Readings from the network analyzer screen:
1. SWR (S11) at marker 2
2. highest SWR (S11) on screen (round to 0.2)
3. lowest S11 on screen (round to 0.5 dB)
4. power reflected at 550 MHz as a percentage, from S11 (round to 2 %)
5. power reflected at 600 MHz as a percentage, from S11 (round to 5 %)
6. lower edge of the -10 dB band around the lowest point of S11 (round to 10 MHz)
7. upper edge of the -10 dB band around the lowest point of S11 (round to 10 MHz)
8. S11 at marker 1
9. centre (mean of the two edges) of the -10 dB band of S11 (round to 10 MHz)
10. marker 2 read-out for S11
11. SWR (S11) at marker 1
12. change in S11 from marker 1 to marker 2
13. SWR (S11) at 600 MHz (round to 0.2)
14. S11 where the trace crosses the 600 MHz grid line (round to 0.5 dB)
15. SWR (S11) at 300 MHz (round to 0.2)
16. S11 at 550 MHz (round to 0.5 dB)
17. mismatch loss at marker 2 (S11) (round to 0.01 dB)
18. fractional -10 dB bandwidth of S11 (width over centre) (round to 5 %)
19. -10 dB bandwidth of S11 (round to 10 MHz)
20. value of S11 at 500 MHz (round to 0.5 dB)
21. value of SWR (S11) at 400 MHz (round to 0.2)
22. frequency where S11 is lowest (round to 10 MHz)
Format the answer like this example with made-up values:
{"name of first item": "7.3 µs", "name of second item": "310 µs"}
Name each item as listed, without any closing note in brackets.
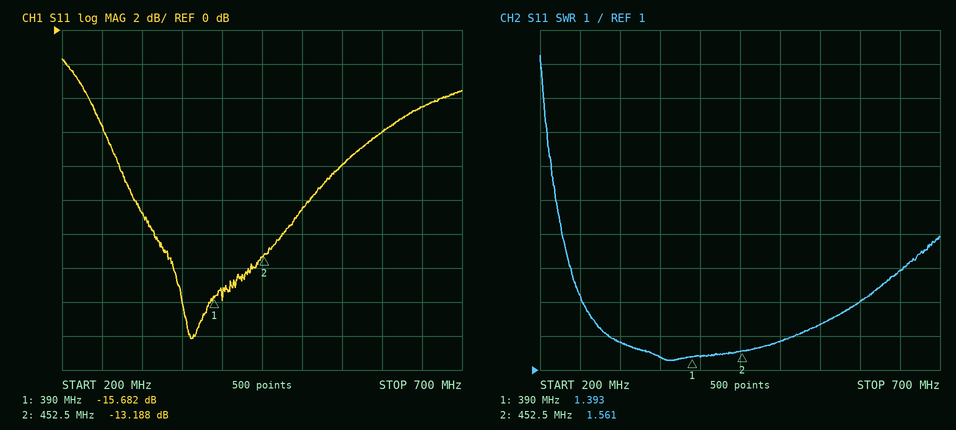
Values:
{"SWR (S11) at marker 2": "1.561", "highest SWR (S11) on screen": "10.2", "lowest S11 on screen": "-18.0 dB", "power reflected at 550 MHz as a percentage, from S11": "16 %", "power reflected at 600 MHz as a percentage, from S11": "25 %", "lower edge of the -10 dB band around the lowest point of S11": "290 MHz", "upper edge of the -10 dB band around the lowest point of S11": "510 MHz", "S11 at marker 1": "-15.682 dB", "centre (mean of the two edges) of the -10 dB band of S11": "400 MHz", "marker 2 read-out for S11": "-13.188 dB", "SWR (S11) at marker 1": "1.393", "change in S11 from marker 1 to marker 2": "2.494 dB", "SWR (S11) at 600 MHz": "3.0", "S11 where the trace crosses the 600 MHz grid line": "-6.0 dB", "SWR (S11) at 300 MHz": "1.8", "S11 at 550 MHz": "-8.0 dB", "mismatch loss at marker 2 (S11)": "0.21 dB", "fractional -10 dB bandwidth of S11 (width over centre)": "55 %", "-10 dB bandwidth of S11": "220 MHz", "value of S11 at 500 MHz": "-10.5 dB", "value of SWR (S11) at 400 MHz": "1.4", "frequency where S11 is lowest": "360 MHz"}
